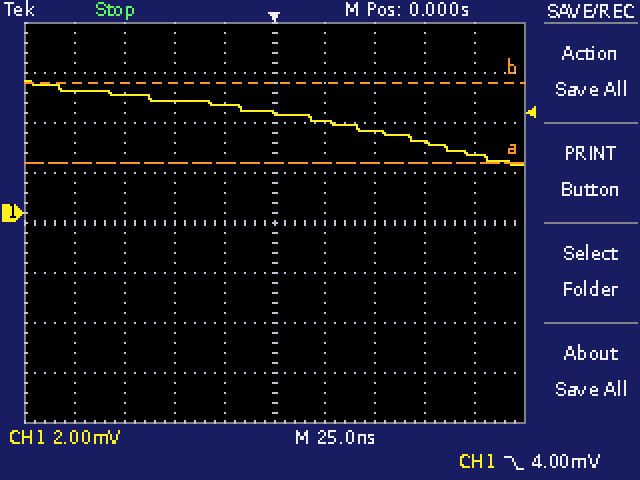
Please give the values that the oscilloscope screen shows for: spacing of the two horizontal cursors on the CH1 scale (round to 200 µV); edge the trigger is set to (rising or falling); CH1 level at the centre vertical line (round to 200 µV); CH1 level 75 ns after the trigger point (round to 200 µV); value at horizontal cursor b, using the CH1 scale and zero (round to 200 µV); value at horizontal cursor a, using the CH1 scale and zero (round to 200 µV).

3.2 mV
falling
4.0 mV
2.8 mV
5.2 mV
2.0 mV
